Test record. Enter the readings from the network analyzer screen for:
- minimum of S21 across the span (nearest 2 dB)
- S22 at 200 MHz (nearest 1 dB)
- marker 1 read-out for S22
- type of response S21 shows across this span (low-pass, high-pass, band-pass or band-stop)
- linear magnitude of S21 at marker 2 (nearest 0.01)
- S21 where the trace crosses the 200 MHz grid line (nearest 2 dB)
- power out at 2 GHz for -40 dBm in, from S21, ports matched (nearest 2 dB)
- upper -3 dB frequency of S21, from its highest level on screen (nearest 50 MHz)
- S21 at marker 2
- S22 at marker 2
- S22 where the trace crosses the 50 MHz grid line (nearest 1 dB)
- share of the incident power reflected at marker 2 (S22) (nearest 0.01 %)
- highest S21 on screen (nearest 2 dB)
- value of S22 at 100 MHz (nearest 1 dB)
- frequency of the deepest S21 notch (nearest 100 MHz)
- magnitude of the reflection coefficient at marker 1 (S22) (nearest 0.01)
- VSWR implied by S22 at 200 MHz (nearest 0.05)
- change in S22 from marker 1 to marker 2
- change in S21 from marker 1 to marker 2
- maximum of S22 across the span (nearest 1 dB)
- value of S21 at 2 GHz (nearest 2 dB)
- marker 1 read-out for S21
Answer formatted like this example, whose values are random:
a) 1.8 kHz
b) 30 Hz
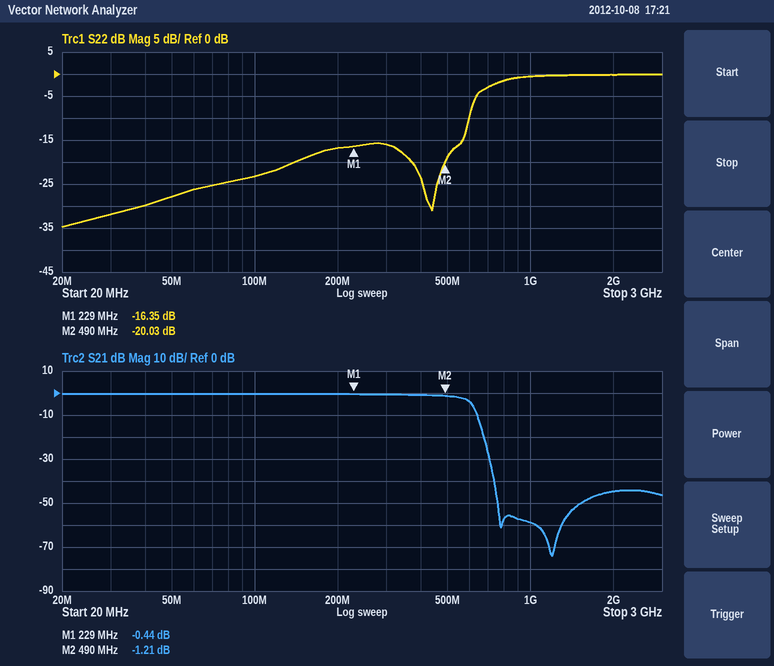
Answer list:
a) -74 dB
b) -17 dB
c) -16.35 dB
d) low-pass
e) 0.87
f) 0 dB
g) -84 dBm
h) 600 MHz
i) -1.21 dB
j) -20.03 dB
k) -28 dB
l) 0.99 %
m) 0 dB
n) -23 dB
o) 1.2 GHz
p) 0.15
q) 1.35
r) -3.68 dB
s) -0.77 dB
t) 0 dB
u) -44 dB
v) -0.44 dB
